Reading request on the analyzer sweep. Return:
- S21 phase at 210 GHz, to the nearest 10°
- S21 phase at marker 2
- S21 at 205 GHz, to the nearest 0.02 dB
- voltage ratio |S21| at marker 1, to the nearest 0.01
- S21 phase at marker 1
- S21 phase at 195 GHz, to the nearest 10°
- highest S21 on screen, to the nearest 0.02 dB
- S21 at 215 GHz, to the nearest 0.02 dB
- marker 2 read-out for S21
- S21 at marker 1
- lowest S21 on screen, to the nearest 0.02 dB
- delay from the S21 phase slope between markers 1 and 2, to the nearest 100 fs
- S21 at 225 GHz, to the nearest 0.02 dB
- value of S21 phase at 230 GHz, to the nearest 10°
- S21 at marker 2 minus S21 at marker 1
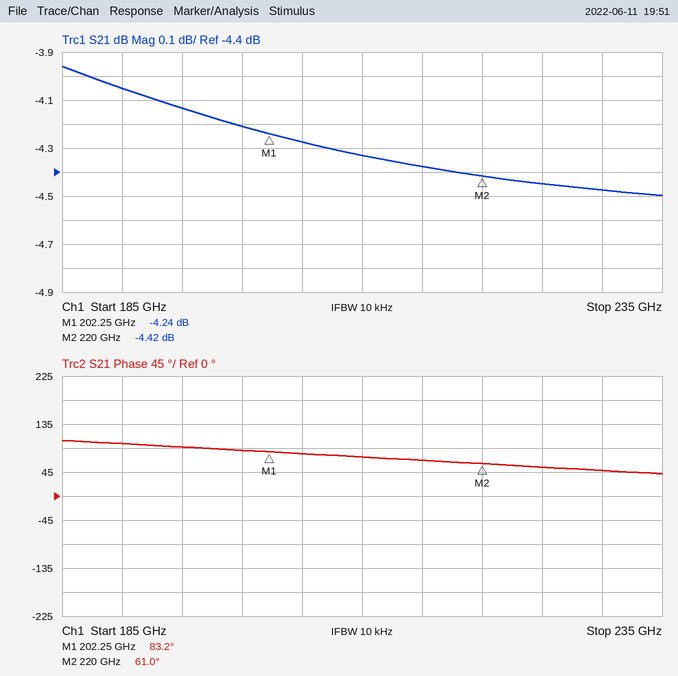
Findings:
70°
61.0°
-4.28 dB
0.61
83.2°
90°
-3.96 dB
-4.38 dB
-4.42 dB
-4.24 dB
-4.50 dB
3.5 ps
-4.44 dB
50°
-0.18 dB
